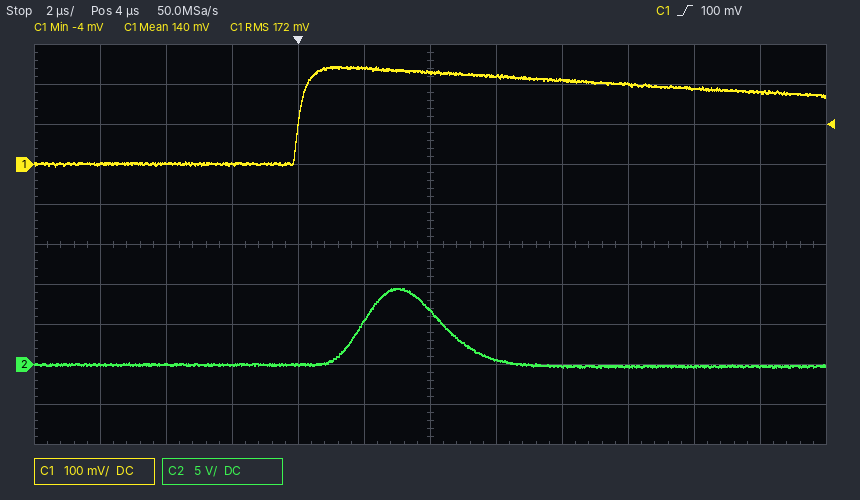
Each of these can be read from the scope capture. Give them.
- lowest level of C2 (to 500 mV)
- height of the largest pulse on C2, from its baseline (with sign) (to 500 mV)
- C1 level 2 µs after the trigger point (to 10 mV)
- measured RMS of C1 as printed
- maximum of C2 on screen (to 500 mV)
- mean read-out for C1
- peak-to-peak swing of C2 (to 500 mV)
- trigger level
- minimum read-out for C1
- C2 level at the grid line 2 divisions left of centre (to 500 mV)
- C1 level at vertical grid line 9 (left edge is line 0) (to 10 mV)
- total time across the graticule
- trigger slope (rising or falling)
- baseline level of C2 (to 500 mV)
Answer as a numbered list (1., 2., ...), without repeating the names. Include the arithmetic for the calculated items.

1. -500 mV
2. 9.5 V − (0.0 V) = +9.5 V
3. 240 mV
4. 172 mV
5. 9.5 V
6. 140 mV
7. 9.5 V − (-500 mV) = 10.0 V
8. 100 mV
9. -4 mV
10. 0.0 V
11. 200 mV
12. 24 µs
13. rising
14. 0.0 V
